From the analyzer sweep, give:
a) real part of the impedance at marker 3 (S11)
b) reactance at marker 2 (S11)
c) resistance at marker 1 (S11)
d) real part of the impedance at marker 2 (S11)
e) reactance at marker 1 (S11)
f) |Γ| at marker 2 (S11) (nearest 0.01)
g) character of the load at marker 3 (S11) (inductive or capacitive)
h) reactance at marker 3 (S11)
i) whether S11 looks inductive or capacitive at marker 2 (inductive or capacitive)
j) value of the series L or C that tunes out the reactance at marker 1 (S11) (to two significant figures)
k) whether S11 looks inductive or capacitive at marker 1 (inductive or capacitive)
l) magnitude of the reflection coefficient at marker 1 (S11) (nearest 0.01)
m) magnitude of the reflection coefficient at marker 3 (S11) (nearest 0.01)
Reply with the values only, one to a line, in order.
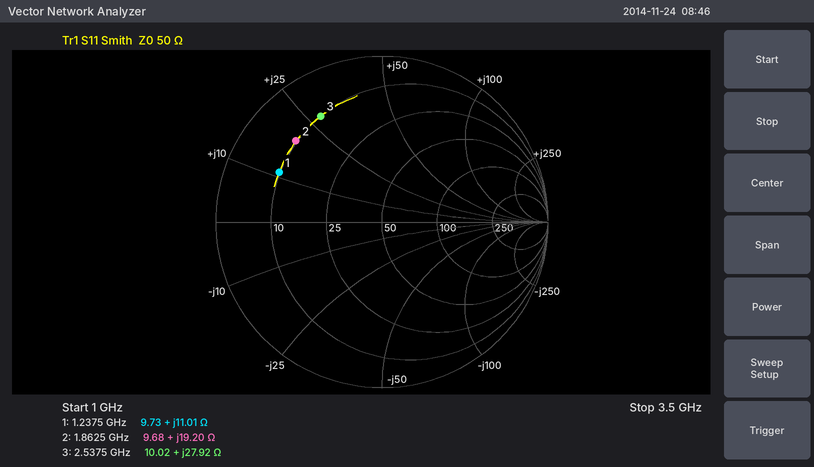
10.02 Ω
+19.20 Ω
9.73 Ω
9.68 Ω
+11.01 Ω
0.71
inductive
+27.92 Ω
inductive
12 pF
inductive
0.69
0.74
